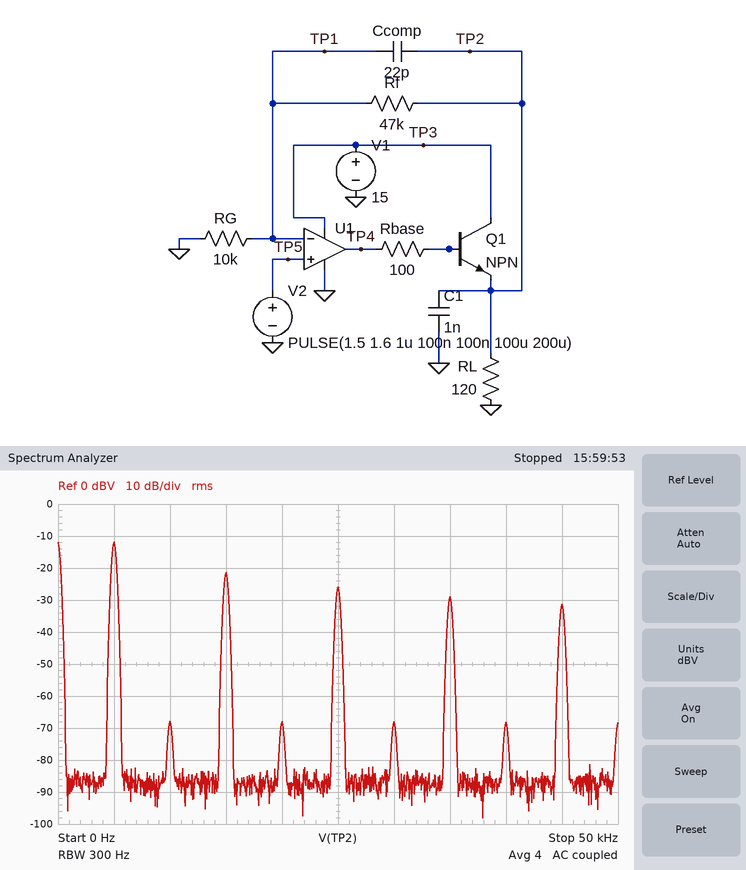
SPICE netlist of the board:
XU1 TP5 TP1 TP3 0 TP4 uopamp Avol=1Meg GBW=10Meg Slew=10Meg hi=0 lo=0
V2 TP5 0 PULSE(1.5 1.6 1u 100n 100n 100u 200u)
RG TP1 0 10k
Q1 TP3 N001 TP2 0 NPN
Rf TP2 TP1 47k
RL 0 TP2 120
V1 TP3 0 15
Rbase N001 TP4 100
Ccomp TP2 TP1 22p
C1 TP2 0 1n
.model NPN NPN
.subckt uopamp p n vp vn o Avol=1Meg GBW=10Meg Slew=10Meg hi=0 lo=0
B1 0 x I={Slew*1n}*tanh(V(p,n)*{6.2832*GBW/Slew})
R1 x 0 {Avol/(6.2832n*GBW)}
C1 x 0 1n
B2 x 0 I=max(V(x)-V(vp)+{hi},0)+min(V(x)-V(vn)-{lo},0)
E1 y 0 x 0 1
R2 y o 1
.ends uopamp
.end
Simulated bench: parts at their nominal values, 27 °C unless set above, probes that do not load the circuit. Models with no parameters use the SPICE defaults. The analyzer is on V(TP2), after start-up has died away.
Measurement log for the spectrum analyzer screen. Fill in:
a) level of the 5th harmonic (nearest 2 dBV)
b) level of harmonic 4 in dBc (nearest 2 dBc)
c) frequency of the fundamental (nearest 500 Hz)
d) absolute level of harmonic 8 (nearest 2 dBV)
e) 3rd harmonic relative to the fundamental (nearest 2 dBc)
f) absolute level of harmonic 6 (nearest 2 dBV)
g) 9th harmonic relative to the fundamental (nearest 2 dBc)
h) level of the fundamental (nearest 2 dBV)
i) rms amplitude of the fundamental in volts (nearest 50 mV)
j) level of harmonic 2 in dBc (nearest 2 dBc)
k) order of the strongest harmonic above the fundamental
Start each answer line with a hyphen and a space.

- -26 dBV
- -56 dBc
- 5.0 kHz
- -68 dBV
- -10 dBc
- -68 dBV
- -20 dBc
- -12 dBV
- 250 mV
- -56 dBc
- 3
